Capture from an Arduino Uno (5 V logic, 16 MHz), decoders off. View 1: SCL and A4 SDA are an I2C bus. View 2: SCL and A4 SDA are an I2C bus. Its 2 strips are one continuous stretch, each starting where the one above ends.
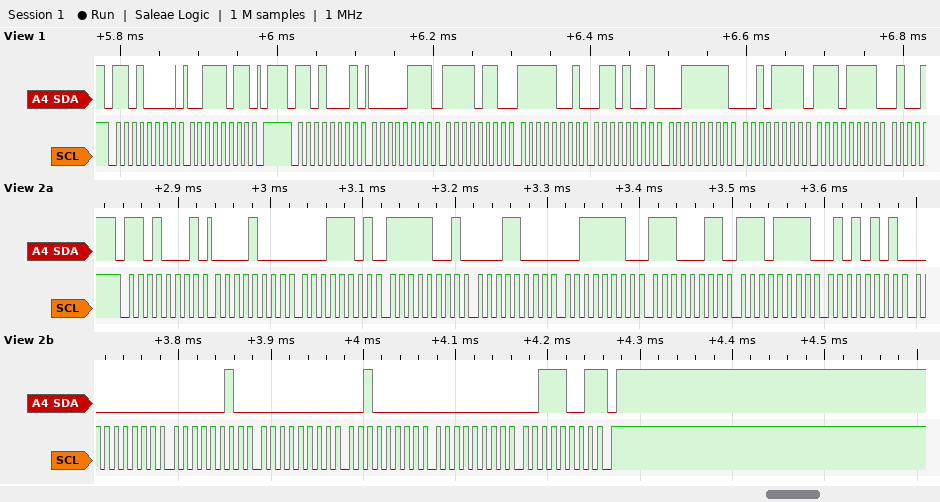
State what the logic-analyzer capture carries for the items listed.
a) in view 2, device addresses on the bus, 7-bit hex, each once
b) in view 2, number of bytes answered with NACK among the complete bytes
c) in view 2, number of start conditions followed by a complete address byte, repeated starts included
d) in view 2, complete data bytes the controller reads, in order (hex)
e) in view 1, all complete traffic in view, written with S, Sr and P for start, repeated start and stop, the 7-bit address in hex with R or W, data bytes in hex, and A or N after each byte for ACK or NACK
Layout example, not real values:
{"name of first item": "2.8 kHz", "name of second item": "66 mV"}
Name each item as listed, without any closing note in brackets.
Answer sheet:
{"in view 2, device addresses on the bus, 7-bit hex, each once": "0x68", "in view 2, number of bytes answered with NACK among the complete bytes": "1", "in view 2, number of start conditions followed by a complete address byte, repeated starts included": "1", "in view 2, complete data bytes the controller reads, in order": "08 1D F9 18 3E E3 EF 55 00 02 00 20 00 39", "in view 1, all complete traffic in view, written with S, Sr and P for start, repeated start and stop, the 7-bit address in hex with R or W, data bytes in hex, and A or N after each byte for ACK or NACK": "S 68W A 3B A P S 68R A 07 A F6 A F9 A 69 A 3F A 2F A EF A"}
